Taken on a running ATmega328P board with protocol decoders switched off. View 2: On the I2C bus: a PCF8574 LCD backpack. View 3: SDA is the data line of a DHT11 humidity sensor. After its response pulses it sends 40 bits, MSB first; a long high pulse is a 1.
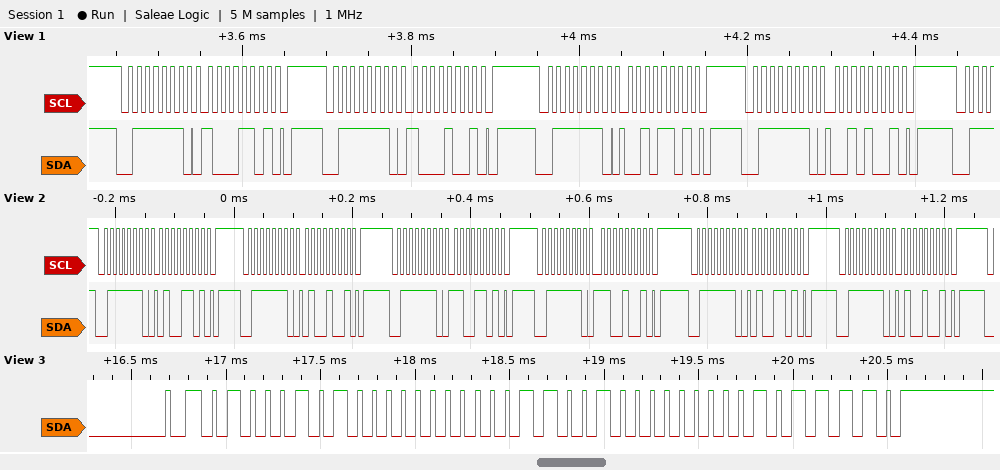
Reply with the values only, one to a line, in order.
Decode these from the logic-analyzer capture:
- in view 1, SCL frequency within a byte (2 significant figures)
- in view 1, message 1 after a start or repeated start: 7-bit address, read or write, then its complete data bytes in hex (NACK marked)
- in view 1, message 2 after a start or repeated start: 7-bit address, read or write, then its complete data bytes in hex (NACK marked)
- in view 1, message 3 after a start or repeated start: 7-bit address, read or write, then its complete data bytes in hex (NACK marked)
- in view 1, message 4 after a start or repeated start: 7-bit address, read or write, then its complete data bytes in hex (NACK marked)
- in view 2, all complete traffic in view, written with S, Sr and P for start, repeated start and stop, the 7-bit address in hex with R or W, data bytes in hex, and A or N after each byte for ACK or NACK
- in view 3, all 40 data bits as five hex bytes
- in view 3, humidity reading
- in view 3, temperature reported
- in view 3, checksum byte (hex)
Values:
100 kHz
0x3F write: 8D
0x3F write: 89
0x3F write: 2D
0x3F write: 29
S 3FW A 4D A P S 3FW A 49 A P S 3FW A CD A P S 3FW A C9 A P S 3FW A 4D A P S 3FW A 49 A P
45 00 19 00 5E
69 %
25.0 °C
0x5E
